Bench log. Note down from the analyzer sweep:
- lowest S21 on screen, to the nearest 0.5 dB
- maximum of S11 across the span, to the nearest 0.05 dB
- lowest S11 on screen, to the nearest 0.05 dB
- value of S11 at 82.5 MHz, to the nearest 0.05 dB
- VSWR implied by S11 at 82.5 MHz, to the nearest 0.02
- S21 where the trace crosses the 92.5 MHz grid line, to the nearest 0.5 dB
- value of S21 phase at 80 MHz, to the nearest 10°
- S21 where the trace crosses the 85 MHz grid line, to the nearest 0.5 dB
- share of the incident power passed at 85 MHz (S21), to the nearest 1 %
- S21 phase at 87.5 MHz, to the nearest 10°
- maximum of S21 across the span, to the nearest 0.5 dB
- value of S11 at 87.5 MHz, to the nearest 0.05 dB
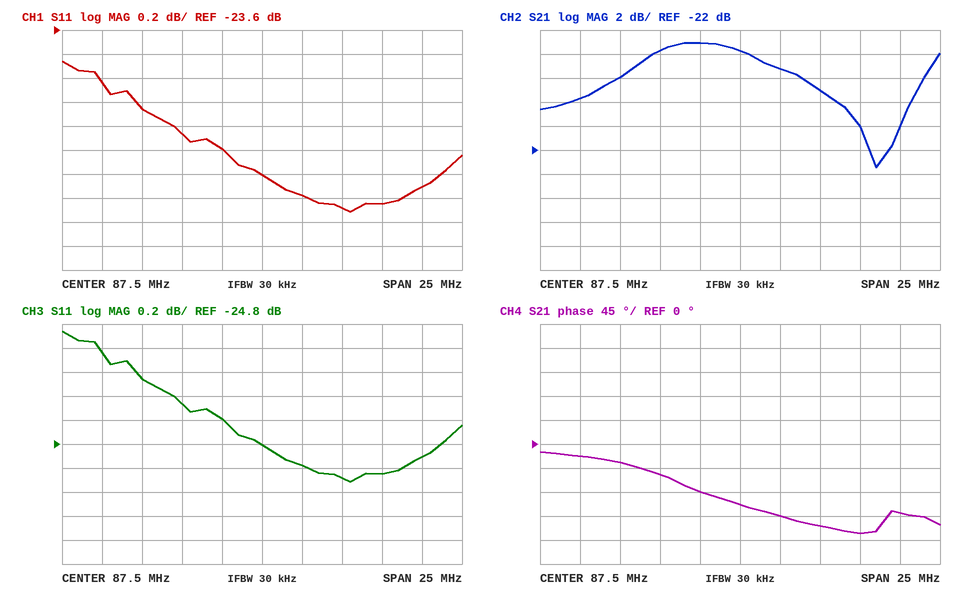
-23.5 dB
-23.85 dB
-25.10 dB
-24.45 dB
1.12
-17.0 dB
-30°
-13.0 dB
5 %
-110°
-13.0 dB
-24.80 dB
